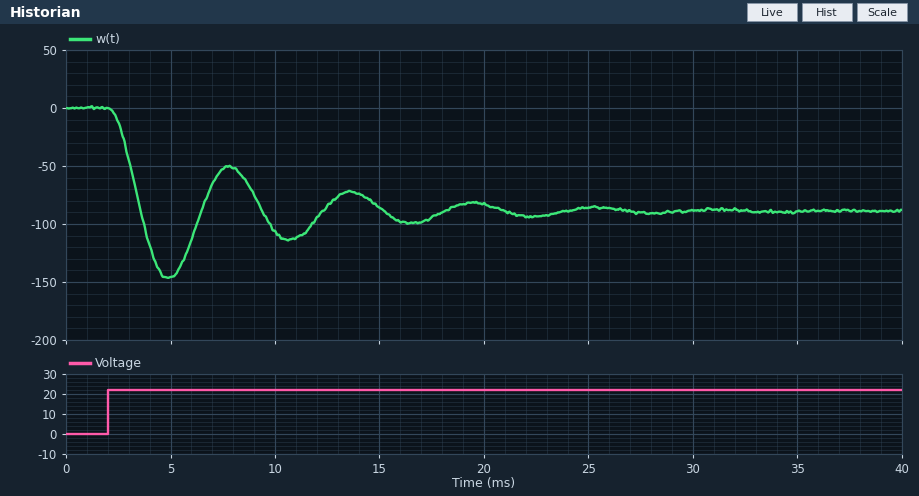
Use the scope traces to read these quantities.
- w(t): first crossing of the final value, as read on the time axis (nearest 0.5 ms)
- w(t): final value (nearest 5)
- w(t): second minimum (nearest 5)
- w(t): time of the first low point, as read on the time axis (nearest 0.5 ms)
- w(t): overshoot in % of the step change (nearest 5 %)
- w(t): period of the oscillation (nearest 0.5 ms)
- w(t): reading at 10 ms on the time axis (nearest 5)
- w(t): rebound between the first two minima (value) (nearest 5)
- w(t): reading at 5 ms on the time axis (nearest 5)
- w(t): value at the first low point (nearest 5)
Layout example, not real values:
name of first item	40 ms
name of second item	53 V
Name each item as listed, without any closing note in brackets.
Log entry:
w(t): first crossing of the final value, as read on the time axis	3.5 ms
w(t): final value	-90
w(t): second minimum	-115
w(t): time of the first low point, as read on the time axis	5.0 ms
w(t): overshoot in % of the step change	65 %
w(t): period of the oscillation	6.0 ms
w(t): reading at 10 ms on the time axis	-105
w(t): rebound between the first two minima (value)	-50
w(t): reading at 5 ms on the time axis	-145
w(t): value at the first low point	-145
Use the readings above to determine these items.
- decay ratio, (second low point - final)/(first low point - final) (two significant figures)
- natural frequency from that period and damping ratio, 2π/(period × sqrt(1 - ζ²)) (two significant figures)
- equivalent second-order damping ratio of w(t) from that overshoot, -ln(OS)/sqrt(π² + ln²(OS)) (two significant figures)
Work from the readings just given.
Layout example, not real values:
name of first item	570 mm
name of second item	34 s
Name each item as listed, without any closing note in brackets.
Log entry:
decay ratio, (second low point - final)/(first low point - final)	0.45
natural frequency from that period and damping ratio, 2π/(period × sqrt(1 - ζ²))	1.1 rad/ms
equivalent second-order damping ratio of w(t) from that overshoot, -ln(OS)/sqrt(π² + ln²(OS))	0.14
